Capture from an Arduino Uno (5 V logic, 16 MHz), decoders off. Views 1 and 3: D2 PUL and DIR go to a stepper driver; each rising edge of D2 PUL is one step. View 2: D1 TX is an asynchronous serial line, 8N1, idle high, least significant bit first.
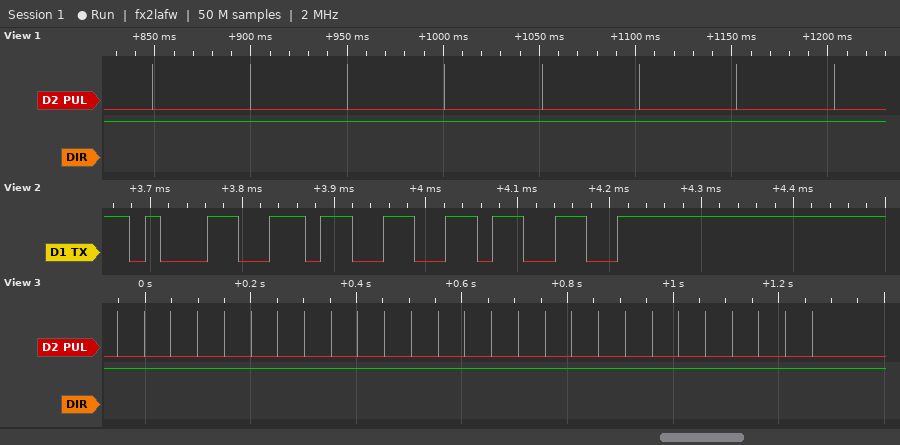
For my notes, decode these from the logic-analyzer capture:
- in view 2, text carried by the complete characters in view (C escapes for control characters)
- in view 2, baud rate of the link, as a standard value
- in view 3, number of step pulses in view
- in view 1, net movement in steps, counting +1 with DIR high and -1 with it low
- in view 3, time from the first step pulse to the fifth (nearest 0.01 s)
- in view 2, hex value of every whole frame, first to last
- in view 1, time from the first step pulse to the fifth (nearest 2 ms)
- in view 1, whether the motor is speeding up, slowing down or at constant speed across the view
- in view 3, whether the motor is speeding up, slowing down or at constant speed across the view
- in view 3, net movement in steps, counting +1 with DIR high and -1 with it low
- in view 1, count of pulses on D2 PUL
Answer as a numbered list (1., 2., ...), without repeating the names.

1. "133"
2. 57600 baud
3. 27
4. +8
5. 0.20 s
6. 0x31 0x33 0x33
7. 202 ms
8. constant speed
9. constant speed
10. +27
11. 8
